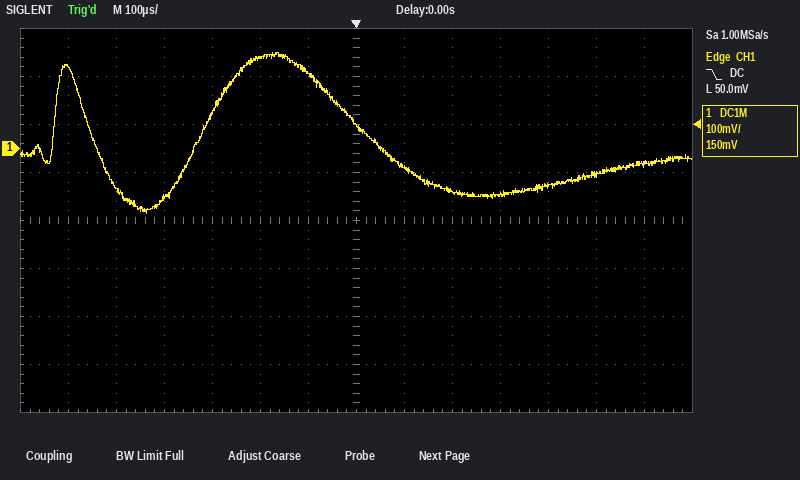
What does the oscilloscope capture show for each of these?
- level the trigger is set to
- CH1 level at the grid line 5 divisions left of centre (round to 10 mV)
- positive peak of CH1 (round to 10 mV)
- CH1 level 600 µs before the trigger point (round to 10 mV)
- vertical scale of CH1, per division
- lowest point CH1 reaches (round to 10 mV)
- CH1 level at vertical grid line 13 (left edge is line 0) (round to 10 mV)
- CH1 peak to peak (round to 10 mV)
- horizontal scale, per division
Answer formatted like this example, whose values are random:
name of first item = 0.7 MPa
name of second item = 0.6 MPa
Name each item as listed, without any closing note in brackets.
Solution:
level the trigger is set to = 50.0 mV
CH1 level at the grid line 5 divisions left of centre = -80 mV
positive peak of CH1 = 200 mV
CH1 level 600 µs before the trigger point = 170 mV
vertical scale of CH1, per division = 100 mV
lowest point CH1 reaches = -140 mV
CH1 level at vertical grid line 13 (left edge is line 0) = -30 mV
CH1 peak to peak = 340 mV
horizontal scale, per division = 100 µs
